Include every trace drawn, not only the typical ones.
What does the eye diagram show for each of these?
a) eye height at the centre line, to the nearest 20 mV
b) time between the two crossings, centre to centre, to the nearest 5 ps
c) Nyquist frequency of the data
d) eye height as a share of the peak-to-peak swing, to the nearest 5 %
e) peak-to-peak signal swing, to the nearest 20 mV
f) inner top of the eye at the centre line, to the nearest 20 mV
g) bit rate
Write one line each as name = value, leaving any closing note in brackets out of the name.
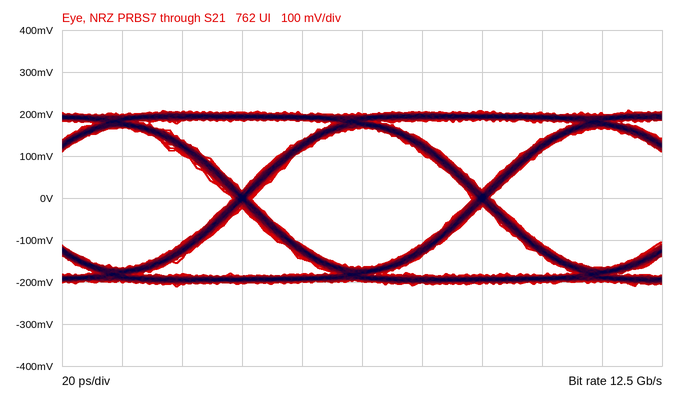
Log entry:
eye height at the centre line, to the nearest 20 mV = 340 mV
time between the two crossings, centre to centre, to the nearest 5 ps = 80 ps
Nyquist frequency of the data = 6.25 GHz
eye height as a share of the peak-to-peak swing, to the nearest 5 % = 80 %
peak-to-peak signal swing, to the nearest 20 mV = 420 mV
inner top of the eye at the centre line, to the nearest 20 mV = 160 mV
bit rate = 12.5 Gb/s
